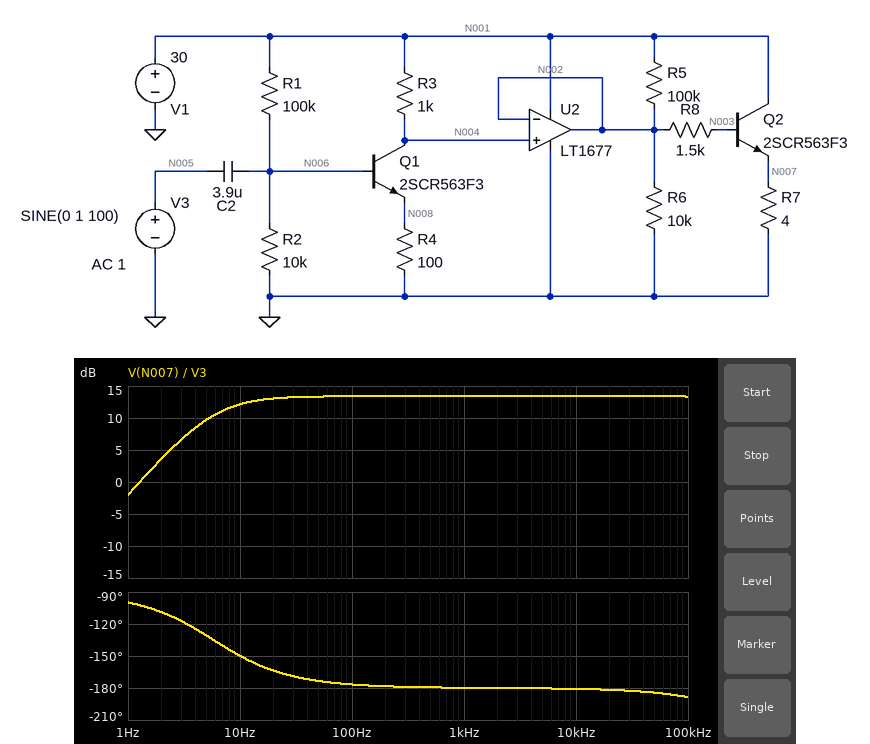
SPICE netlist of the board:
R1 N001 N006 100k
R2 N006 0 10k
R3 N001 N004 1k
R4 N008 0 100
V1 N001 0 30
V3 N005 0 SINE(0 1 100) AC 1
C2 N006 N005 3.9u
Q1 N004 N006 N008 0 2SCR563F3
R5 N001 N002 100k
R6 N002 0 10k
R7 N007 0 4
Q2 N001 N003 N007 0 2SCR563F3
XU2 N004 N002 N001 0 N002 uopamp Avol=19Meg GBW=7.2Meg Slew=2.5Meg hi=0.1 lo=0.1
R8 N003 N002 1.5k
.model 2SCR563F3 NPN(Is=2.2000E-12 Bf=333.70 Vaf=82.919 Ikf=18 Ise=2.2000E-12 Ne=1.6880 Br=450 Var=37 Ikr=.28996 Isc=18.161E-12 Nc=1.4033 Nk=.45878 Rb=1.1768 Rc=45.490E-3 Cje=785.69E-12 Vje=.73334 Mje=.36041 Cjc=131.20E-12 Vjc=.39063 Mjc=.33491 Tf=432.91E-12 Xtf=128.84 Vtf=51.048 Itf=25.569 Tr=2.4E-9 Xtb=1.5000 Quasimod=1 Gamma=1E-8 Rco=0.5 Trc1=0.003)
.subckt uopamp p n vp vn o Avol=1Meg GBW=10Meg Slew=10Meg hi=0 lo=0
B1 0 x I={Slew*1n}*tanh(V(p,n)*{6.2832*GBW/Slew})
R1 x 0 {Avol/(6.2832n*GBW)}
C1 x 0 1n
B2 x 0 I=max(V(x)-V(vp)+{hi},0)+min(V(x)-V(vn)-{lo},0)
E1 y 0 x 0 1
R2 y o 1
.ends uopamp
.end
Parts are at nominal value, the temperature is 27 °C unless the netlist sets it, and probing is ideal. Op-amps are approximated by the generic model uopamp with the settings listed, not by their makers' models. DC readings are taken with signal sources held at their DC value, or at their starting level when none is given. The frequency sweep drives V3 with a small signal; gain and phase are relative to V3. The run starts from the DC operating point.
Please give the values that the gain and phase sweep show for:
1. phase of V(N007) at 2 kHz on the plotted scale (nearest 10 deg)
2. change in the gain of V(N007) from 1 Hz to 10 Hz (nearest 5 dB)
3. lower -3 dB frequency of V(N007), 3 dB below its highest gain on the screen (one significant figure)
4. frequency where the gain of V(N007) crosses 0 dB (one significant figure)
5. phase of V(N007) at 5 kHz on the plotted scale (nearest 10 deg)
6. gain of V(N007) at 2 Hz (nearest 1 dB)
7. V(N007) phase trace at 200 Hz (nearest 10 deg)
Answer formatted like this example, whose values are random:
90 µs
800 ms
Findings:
-180 deg
15 dB
6 Hz
1 Hz
-180 deg
4 dB
-180 deg
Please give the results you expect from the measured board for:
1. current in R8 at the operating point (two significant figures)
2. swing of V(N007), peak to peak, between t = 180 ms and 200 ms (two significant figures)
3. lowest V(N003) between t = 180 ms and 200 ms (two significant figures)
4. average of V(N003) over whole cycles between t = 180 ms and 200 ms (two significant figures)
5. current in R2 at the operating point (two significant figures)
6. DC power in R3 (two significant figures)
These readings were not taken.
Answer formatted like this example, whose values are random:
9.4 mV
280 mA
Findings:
4.0 mA
9.3 V
2.1 V
6.9 V
230 µA
290 mW
